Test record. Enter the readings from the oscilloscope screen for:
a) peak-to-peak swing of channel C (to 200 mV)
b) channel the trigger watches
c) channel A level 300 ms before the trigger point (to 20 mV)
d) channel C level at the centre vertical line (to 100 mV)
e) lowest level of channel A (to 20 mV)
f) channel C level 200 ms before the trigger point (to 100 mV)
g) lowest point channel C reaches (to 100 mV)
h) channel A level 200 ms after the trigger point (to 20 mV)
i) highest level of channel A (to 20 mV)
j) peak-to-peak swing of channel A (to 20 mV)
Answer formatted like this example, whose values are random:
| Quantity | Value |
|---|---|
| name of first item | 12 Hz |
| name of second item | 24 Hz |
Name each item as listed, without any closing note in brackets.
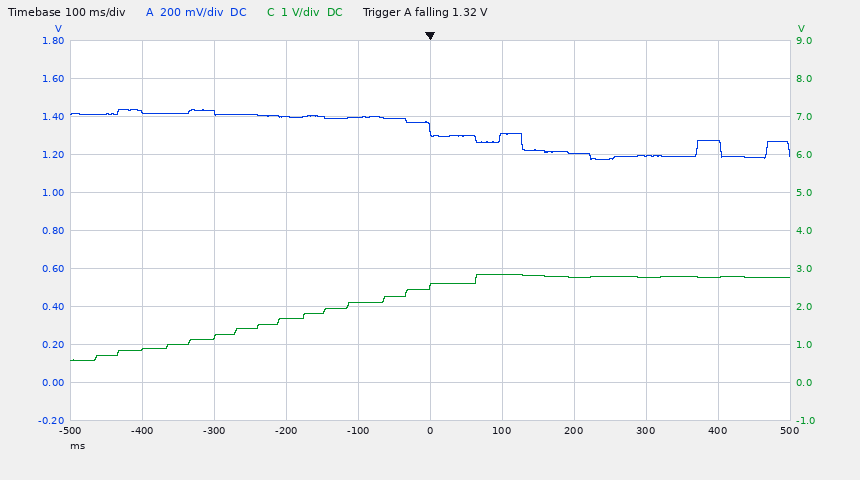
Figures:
| Quantity | Value |
|---|---|
| peak-to-peak swing of channel C | 2.2 V |
| channel the trigger watches | channel A |
| channel A level 300 ms before the trigger point | 1.42 V |
| channel C level at the centre vertical line | 2.5 V |
| lowest level of channel A | 1.18 V |
| channel C level 200 ms before the trigger point | 1.7 V |
| lowest point channel C reaches | 600 mV |
| channel A level 200 ms after the trigger point | 1.20 V |
| highest level of channel A | 1.44 V |
| peak-to-peak swing of channel A | 260 mV |
